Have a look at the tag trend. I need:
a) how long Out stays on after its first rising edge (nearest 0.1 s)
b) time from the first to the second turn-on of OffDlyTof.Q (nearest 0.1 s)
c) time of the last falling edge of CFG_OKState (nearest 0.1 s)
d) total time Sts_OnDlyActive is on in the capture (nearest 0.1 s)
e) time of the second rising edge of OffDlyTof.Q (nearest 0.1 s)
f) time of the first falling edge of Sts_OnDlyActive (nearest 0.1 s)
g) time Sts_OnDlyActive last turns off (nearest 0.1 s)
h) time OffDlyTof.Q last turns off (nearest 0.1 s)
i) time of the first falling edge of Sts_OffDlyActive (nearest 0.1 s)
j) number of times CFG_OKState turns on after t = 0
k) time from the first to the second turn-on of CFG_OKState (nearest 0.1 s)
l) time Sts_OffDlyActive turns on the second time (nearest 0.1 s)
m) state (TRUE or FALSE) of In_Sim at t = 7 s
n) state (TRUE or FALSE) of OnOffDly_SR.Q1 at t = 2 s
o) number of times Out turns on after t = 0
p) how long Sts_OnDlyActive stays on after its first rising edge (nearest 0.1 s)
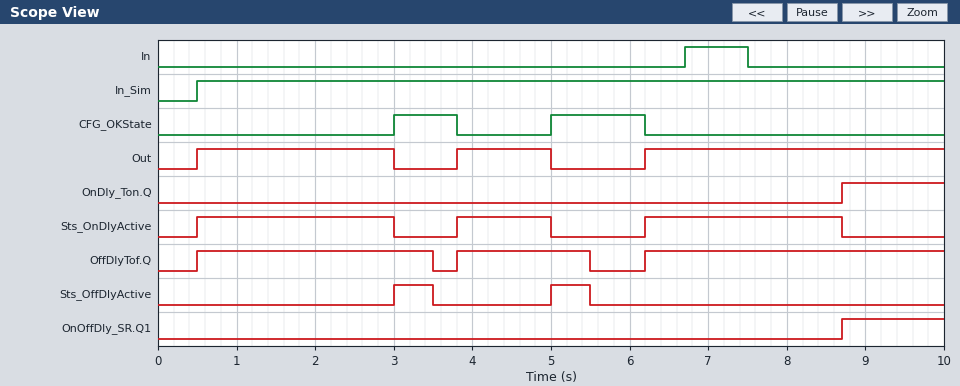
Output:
2.5 s
3.3 s
6.2 s
6.2 s
3.8 s
3.0 s
8.7 s
5.5 s
3.5 s
2
2.0 s
5.0 s
TRUE
FALSE
3
2.5 s
